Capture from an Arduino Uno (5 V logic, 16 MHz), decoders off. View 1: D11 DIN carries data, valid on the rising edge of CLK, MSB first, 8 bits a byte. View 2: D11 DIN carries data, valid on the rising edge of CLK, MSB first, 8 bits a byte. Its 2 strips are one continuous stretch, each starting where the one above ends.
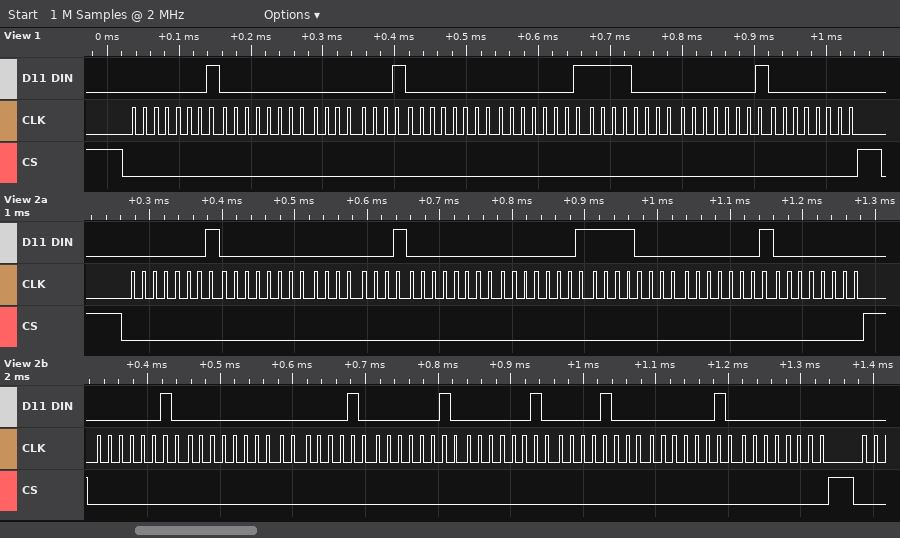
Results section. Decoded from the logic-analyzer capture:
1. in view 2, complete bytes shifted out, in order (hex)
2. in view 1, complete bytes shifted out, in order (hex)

01 00 01 00 01 F0 01 00 02 00 02 02 02 08 02 00
0x01 0x00 0x01 0x00 0x01 0xF0 0x01 0x00
